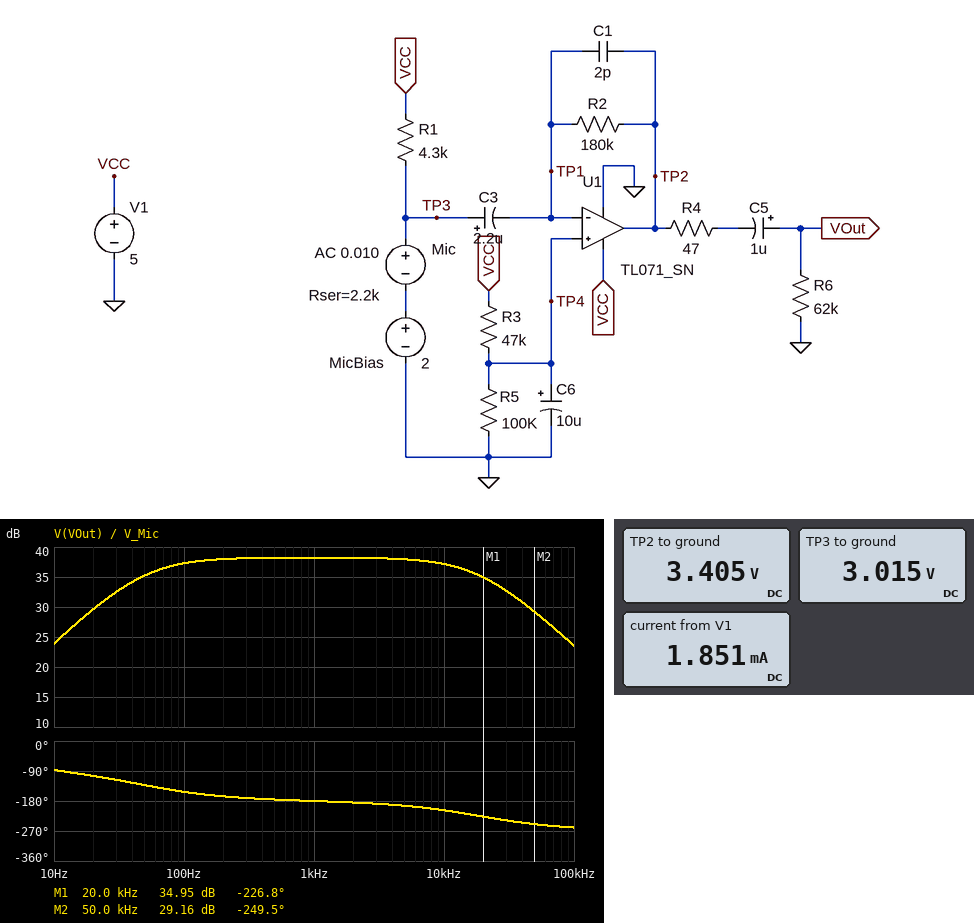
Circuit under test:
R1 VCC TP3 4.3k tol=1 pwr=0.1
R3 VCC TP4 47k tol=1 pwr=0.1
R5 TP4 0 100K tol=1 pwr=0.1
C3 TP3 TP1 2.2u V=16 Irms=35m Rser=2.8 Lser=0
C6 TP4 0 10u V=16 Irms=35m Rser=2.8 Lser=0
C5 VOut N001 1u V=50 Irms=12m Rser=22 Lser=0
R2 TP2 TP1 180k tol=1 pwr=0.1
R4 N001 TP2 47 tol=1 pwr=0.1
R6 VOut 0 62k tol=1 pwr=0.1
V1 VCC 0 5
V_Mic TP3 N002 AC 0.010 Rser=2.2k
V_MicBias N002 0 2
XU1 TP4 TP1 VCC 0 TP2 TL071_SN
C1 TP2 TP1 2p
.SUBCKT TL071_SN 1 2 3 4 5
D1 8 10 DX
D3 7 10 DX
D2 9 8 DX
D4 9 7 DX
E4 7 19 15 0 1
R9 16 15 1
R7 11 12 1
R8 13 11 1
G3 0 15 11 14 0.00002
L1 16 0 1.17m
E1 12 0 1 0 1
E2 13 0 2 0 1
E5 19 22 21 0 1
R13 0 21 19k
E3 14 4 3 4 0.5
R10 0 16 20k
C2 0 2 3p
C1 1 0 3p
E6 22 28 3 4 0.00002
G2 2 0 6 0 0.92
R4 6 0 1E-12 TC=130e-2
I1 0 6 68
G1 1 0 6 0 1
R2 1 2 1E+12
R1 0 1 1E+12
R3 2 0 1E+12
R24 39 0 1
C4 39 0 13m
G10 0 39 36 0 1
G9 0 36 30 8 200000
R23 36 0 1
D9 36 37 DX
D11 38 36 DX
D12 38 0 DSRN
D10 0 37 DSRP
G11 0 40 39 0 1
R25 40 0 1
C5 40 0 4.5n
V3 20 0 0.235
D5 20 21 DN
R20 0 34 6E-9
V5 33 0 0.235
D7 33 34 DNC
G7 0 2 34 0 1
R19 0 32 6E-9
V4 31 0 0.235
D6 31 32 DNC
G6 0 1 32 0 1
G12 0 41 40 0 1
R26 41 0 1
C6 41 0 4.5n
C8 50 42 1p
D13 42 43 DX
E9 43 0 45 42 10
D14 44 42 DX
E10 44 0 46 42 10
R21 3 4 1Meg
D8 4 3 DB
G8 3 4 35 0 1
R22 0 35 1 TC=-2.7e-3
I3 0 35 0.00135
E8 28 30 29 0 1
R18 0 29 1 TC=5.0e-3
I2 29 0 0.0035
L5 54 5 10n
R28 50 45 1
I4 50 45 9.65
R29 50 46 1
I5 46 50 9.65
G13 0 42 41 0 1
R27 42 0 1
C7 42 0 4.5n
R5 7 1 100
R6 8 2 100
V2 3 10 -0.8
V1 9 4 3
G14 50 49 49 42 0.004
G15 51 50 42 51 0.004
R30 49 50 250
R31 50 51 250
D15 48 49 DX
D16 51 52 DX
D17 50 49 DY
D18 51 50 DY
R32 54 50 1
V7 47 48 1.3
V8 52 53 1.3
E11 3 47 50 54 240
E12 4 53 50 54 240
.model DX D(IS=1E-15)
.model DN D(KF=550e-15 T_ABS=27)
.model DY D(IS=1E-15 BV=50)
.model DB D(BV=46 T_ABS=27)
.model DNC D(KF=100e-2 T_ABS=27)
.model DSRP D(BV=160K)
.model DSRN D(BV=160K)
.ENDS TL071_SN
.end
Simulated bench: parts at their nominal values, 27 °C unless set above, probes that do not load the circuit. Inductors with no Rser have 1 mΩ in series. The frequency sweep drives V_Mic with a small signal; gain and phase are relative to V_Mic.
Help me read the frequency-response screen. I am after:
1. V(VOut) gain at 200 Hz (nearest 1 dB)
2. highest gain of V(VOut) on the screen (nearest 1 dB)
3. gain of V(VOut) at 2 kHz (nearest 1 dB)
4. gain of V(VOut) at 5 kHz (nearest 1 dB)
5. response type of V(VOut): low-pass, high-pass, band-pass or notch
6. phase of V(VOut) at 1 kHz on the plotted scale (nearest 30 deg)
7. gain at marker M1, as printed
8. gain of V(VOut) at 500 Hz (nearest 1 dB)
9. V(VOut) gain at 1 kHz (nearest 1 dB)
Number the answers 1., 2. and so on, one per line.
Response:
1. 38 dB
2. 38 dB
3. 38 dB
4. 38 dB
5. band-pass
6. -180 deg
7. 34.95 dB
8. 38 dB
9. 38 dB
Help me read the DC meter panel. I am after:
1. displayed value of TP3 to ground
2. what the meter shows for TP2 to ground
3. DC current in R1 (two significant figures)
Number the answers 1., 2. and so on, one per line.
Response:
1. 3.015 V
2. 3.405 V
3. 460 µA
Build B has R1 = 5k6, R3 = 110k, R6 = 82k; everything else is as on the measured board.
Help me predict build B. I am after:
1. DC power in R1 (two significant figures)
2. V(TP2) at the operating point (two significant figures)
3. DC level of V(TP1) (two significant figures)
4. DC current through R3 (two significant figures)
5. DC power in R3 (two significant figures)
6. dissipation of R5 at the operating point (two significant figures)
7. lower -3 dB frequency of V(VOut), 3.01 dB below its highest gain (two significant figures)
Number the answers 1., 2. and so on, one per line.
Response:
1. 830 µW
2. 2.2 V
3. 2.5 V
4. 23 µA
5. 59 µW
6. 60 µW
7. 46 Hz
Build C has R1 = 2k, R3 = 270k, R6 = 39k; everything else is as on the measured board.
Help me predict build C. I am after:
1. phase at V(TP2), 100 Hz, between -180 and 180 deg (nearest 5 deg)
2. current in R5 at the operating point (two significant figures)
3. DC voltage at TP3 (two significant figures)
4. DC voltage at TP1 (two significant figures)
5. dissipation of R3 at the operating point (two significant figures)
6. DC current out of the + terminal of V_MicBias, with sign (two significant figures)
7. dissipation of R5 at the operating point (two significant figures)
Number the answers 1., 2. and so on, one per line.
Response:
1. 10 deg
2. 24 µA
3. 3.6 V
4. 2.4 V
5. 25 µW
6. -710 µA
7. 57 µW
